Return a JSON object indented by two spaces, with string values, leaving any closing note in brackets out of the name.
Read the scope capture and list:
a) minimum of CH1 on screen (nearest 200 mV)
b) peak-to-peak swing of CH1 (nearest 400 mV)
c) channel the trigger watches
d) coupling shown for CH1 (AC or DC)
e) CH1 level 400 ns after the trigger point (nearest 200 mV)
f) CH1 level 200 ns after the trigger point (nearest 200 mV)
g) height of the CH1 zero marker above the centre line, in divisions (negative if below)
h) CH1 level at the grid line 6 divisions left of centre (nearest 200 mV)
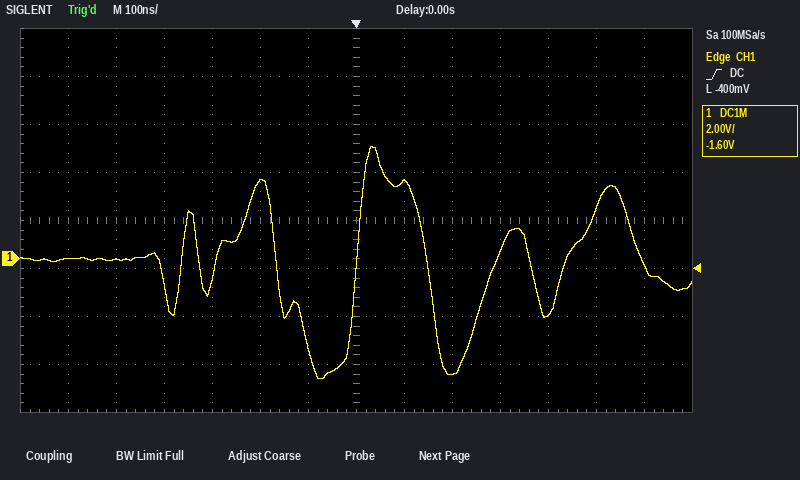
{
  "minimum of CH1 on screen": "-5.0 V",
  "peak-to-peak swing of CH1": "9.6 V",
  "channel the trigger watches": "CH1",
  "coupling shown for CH1": "DC",
  "CH1 level 400 ns after the trigger point": "-2.4 V",
  "CH1 level 200 ns after the trigger point": "-4.8 V",
  "height of the CH1 zero marker above the centre line, in divisions": "-0.8 div",
  "CH1 level at the grid line 6 divisions left of centre": "0.0 V"
}
